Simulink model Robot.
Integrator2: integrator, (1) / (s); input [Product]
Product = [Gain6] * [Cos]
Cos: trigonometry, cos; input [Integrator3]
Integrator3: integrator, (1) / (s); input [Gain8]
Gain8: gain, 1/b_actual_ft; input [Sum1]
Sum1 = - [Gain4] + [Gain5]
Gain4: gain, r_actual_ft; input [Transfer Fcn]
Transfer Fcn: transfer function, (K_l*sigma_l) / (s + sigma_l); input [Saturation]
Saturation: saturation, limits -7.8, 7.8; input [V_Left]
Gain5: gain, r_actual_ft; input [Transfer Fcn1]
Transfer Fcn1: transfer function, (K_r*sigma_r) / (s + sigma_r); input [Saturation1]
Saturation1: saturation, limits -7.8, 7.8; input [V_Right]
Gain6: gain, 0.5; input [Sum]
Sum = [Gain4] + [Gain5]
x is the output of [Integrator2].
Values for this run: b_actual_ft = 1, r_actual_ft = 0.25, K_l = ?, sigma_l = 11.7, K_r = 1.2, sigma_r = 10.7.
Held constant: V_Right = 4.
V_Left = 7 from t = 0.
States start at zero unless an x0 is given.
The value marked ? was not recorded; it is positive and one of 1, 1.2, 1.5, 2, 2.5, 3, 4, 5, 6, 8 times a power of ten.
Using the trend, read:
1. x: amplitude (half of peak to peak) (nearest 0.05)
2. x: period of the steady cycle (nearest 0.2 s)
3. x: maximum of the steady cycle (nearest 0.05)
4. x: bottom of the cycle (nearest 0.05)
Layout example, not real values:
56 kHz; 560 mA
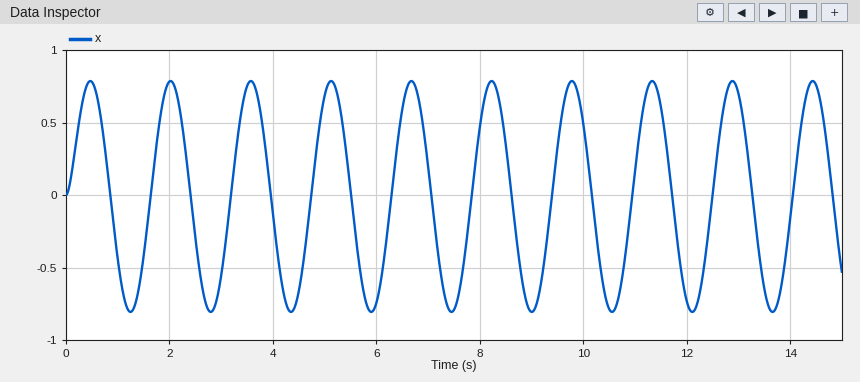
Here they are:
0.80; 1.6 s; 0.80; -0.80
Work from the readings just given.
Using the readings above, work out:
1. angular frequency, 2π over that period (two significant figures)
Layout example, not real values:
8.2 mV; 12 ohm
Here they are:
3.9 rad/s
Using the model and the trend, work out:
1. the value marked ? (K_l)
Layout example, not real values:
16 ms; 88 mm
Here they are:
3
